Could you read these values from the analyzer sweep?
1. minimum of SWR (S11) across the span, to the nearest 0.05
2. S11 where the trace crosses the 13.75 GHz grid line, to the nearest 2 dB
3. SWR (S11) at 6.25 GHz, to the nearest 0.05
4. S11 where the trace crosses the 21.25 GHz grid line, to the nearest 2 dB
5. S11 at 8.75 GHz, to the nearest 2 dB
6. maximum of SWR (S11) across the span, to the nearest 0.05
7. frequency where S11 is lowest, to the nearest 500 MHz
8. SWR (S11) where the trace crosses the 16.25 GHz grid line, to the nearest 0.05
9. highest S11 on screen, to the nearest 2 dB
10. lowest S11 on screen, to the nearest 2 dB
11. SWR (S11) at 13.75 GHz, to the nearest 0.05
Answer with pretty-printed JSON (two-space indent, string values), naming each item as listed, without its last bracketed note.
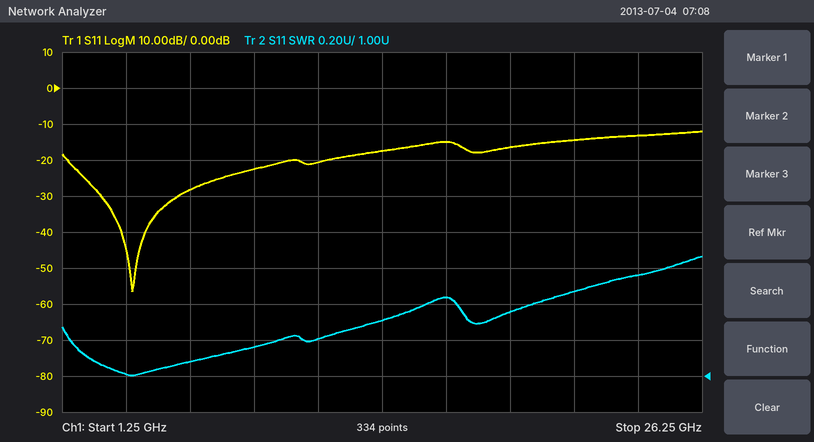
{
  "minimum of SWR (S11) across the span, to the nearest 0.05": "1.00",
  "S11 where the trace crosses the 13.75 GHz grid line, to the nearest 2 dB": "-18 dB",
  "SWR (S11) at 6.25 GHz, to the nearest 0.05": "1.10",
  "S11 where the trace crosses the 21.25 GHz grid line, to the nearest 2 dB": "-14 dB",
  "S11 at 8.75 GHz, to the nearest 2 dB": "-22 dB",
  "maximum of SWR (S11) across the span, to the nearest 0.05": "1.65",
  "frequency where S11 is lowest, to the nearest 500 MHz": "4.0 GHz",
  "SWR (S11) where the trace crosses the 16.25 GHz grid line, to the nearest 0.05": "1.45",
  "highest S11 on screen, to the nearest 2 dB": "-12 dB",
  "lowest S11 on screen, to the nearest 2 dB": "-56 dB",
  "SWR (S11) at 13.75 GHz, to the nearest 0.05": "1.30"
}
